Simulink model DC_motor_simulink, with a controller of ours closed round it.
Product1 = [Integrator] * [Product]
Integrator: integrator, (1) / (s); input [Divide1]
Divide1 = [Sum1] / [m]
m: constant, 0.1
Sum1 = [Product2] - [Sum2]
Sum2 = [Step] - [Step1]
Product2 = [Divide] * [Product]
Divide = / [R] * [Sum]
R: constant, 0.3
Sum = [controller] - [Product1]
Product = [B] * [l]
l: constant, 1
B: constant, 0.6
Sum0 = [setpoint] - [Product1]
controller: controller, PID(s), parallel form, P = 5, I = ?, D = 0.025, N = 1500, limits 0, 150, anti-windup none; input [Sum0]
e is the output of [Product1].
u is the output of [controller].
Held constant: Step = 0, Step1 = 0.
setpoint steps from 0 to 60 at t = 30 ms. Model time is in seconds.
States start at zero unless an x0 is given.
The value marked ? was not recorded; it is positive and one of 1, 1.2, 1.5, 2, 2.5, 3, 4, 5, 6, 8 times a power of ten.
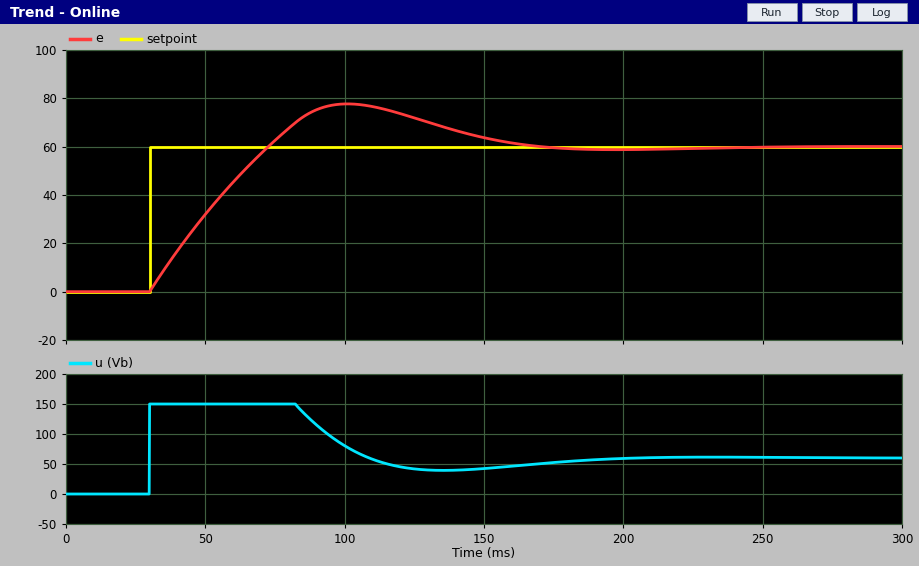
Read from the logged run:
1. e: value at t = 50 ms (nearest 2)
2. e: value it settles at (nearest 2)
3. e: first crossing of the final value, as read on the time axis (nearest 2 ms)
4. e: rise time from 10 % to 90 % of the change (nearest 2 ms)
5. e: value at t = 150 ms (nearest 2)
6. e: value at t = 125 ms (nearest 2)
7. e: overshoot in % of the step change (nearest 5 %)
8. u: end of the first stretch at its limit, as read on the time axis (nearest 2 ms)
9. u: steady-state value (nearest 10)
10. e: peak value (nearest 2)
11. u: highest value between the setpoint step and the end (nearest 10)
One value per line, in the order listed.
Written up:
32
60
72 ms
34 ms
64
72
30 %
82 ms
60
78
150
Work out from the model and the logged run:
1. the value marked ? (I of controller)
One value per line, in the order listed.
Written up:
200
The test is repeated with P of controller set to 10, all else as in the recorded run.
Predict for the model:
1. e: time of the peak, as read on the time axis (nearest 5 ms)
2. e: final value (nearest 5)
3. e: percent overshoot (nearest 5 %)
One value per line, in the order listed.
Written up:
95 ms
60
20 %
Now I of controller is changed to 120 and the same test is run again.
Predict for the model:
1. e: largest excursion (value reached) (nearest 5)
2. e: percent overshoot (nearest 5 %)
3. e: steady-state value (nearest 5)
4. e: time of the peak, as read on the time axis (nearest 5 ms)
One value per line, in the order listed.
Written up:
70
15 %
60
105 ms
